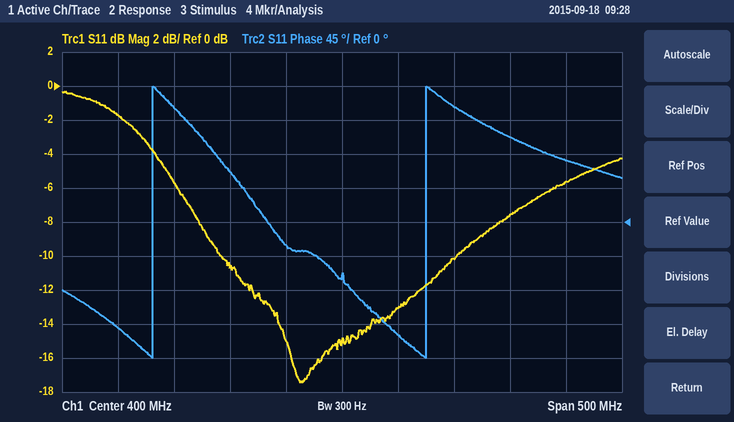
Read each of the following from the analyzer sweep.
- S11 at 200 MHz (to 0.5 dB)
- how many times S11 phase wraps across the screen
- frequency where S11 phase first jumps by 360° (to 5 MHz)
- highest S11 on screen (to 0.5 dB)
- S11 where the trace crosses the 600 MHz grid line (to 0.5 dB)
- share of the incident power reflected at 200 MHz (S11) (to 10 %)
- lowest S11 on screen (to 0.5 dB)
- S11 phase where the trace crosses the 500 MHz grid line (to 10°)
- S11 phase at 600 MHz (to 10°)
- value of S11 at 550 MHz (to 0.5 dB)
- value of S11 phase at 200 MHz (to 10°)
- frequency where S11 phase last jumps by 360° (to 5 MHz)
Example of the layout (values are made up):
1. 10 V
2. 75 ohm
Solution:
1. -1.5 dB
2. 2
3. 230 MHz
4. -0.5 dB
5. -5.5 dB
6. 70 %
7. -17.5 dB
8. 150°
9. 80°
10. -7.5 dB
11. -140°
12. 475 MHz
